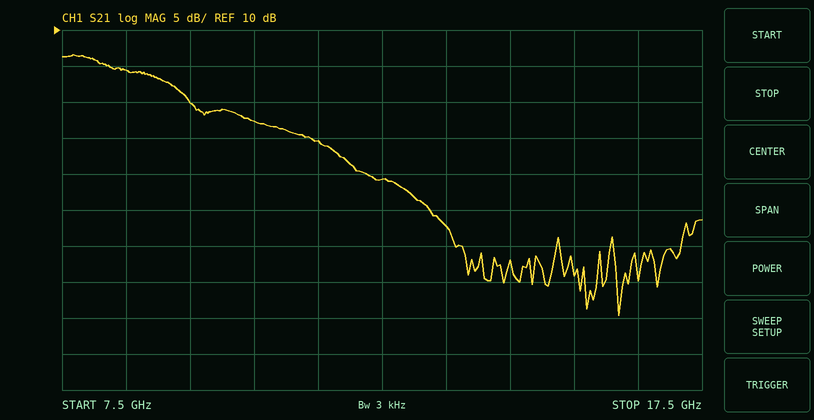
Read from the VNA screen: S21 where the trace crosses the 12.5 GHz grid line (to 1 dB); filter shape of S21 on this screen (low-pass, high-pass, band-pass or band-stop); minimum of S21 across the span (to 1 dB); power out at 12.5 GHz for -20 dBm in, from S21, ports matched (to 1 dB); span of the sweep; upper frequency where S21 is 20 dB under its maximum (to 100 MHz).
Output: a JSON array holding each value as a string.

["-11 dB", "low-pass", "-30 dB", "-31 dBm", "10 GHz", "13.0 GHz"]
